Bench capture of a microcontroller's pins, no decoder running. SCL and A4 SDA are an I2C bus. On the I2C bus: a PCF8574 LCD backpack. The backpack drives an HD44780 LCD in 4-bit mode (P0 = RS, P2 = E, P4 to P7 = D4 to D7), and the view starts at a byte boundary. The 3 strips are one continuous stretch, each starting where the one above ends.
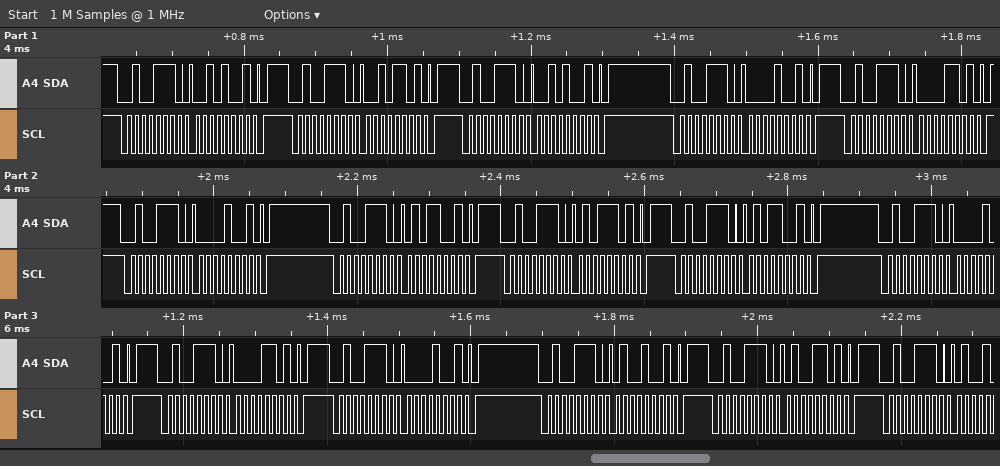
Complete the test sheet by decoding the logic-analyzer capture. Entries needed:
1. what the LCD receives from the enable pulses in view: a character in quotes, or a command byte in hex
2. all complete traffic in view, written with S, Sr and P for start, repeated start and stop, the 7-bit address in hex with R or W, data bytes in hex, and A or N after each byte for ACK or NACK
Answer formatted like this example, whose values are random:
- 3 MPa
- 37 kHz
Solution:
- ' ' 'P'
- S 27W A 29 A P S 27W A 2D A P S 27W A 29 A P S 27W A 09 A P S 27W A 0D A P S 27W A 09 A P S 27W A 59 A P S 27W A 5D A P S 27W A 59 A P S 27W A 09 A P S 27W A 0D A P S 27W A 09 A P S 27W A 49 A P S 27W A 4D A P S 27W A
